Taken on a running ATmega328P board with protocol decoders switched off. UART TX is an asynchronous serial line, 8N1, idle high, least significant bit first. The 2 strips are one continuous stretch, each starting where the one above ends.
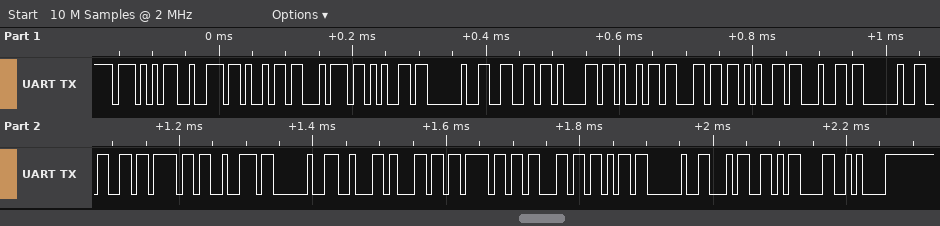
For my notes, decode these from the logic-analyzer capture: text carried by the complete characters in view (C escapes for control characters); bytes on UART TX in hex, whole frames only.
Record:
"Write failed for block 4\r\n"
57 72 69 74 65 20 66 61 69 6C 65 64 20 66 6F 72 20 62 6C 6F 63 6B 20 34 0D 0A
